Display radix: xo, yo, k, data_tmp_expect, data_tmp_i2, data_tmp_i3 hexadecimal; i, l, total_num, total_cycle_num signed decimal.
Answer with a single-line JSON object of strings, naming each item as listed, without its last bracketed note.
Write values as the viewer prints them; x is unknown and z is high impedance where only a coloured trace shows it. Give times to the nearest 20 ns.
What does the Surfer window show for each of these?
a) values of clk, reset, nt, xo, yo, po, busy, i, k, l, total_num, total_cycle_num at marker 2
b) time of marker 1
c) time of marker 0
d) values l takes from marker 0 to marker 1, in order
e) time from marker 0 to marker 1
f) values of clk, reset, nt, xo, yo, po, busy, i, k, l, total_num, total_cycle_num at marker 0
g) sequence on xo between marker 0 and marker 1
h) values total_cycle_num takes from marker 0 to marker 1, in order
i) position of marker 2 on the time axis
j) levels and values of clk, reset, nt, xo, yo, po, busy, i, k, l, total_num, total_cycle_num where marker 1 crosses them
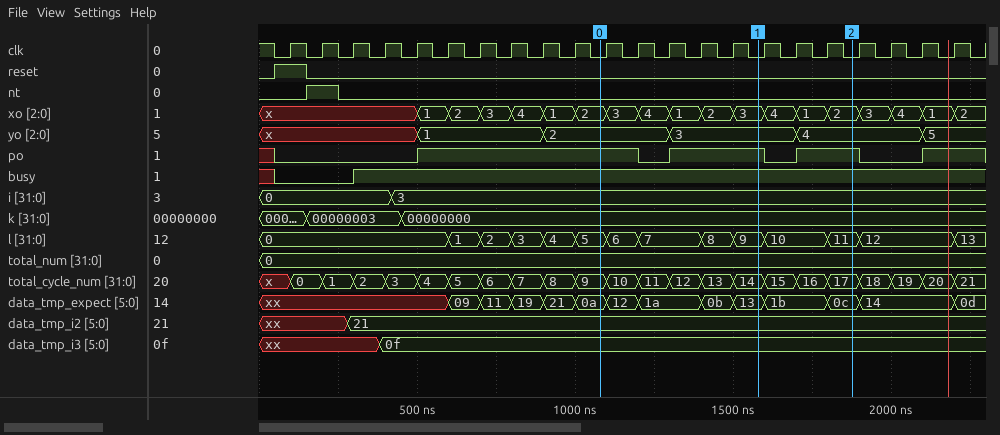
{"values of clk, reset, nt, xo, yo, po, busy, i, k, l, total_num, total_cycle_num at marker 2": "clk=0, reset=0, nt=0, xo=2, yo=4, po=1, busy=1, i=3, k=00000000, l=11, total_num=0, total_cycle_num=17", "time of marker 1": "1580 ns", "time of marker 0": "1080 ns", "values l takes from marker 0 to marker 1, in order": "5, 6, 7, 8, 9", "time from marker 0 to marker 1": "500 ns", "values of clk, reset, nt, xo, yo, po, busy, i, k, l, total_num, total_cycle_num at marker 0": "clk=0, reset=0, nt=0, xo=2, yo=2, po=1, busy=1, i=3, k=00000000, l=5, total_num=0, total_cycle_num=9", "sequence on xo between marker 0 and marker 1": "2, 3, 4, 1, 2, 3", "values total_cycle_num takes from marker 0 to marker 1, in order": "9, 10, 11, 12, 13, 14", "position of marker 2 on the time axis": "1880 ns", "levels and values of clk, reset, nt, xo, yo, po, busy, i, k, l, total_num, total_cycle_num where marker 1 crosses them": "clk=0, reset=0, nt=0, xo=3, yo=3, po=1, busy=1, i=3, k=00000000, l=9, total_num=0, total_cycle_num=14"}
